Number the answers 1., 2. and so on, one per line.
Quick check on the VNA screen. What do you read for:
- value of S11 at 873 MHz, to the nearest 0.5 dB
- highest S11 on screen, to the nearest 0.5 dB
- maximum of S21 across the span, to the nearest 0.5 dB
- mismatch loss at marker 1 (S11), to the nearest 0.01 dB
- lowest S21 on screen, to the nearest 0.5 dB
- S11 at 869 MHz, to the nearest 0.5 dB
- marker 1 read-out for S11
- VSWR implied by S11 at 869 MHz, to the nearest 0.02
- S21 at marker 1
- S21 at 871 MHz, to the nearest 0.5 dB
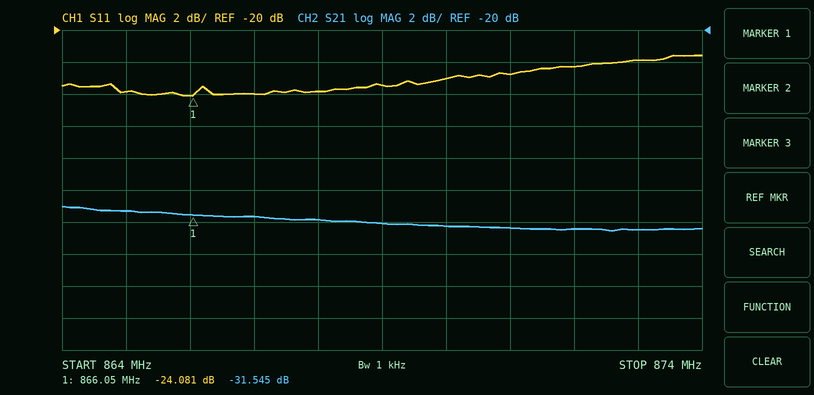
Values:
1. -22.0 dB
2. -21.5 dB
3. -31.0 dB
4. 0.02 dB
5. -32.5 dB
6. -23.5 dB
7. -24.081 dB
8. 1.14
9. -31.545 dB
10. -32.5 dB
